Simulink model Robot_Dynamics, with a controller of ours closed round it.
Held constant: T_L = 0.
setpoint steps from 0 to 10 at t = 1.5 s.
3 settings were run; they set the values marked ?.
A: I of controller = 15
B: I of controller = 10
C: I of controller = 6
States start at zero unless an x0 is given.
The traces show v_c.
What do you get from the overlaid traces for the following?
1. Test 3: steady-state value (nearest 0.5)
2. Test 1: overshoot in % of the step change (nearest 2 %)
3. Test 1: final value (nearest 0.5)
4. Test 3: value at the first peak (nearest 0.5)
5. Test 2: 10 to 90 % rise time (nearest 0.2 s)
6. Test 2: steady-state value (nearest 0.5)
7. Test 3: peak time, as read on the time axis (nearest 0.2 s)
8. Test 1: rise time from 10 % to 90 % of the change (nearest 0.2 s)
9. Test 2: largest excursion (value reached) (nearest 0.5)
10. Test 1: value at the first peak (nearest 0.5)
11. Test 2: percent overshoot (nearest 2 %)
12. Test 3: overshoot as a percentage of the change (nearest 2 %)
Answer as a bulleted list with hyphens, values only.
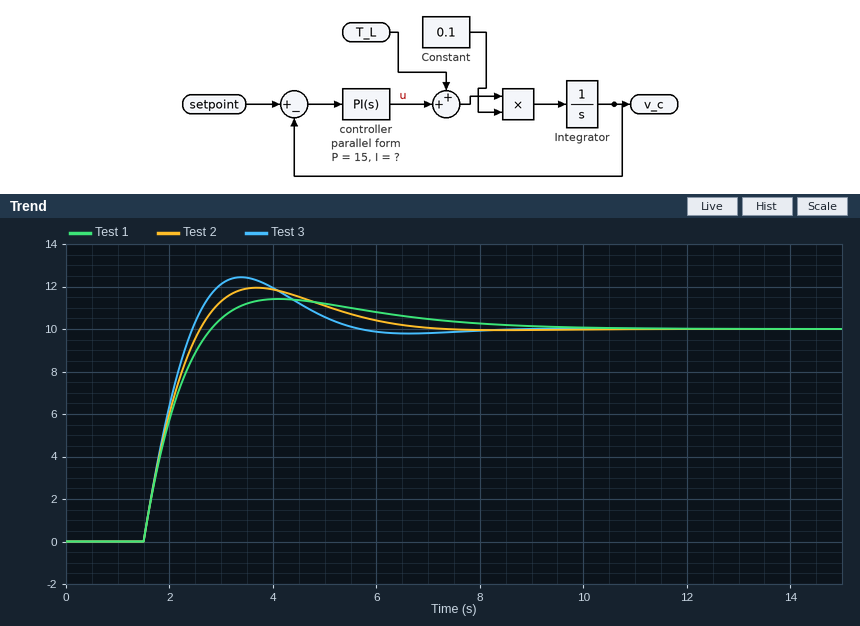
- 10.0
- 14 %
- 10.0
- 12.5
- 0.8 s
- 10.0
- 3.4 s
- 1.0 s
- 12.0
- 11.5
- 20 %
- 24 %
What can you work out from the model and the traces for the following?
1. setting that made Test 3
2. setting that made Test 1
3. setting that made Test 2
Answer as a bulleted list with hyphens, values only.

- A
- C
- B
